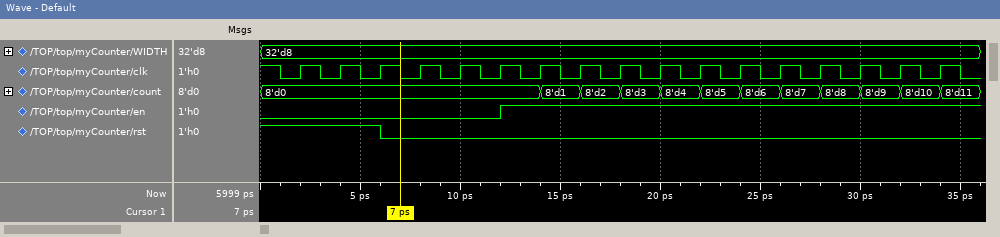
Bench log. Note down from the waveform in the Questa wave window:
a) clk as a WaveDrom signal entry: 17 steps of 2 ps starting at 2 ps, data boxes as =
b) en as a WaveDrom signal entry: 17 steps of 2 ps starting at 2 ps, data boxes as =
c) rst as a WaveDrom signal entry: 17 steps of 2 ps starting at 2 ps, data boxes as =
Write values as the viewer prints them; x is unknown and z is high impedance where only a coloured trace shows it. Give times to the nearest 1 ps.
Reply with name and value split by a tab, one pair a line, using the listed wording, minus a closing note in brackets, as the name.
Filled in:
clk as a WaveDrom signal entry: 17 steps of 2 ps starting at 2 ps, data boxes as =	{name: 'clk', wave: 'p................'}
en as a WaveDrom signal entry: 17 steps of 2 ps starting at 2 ps, data boxes as =	{name: 'en', wave: '0....1...........'}
rst as a WaveDrom signal entry: 17 steps of 2 ps starting at 2 ps, data boxes as =	{name: 'rst', wave: '1.0..............'}
